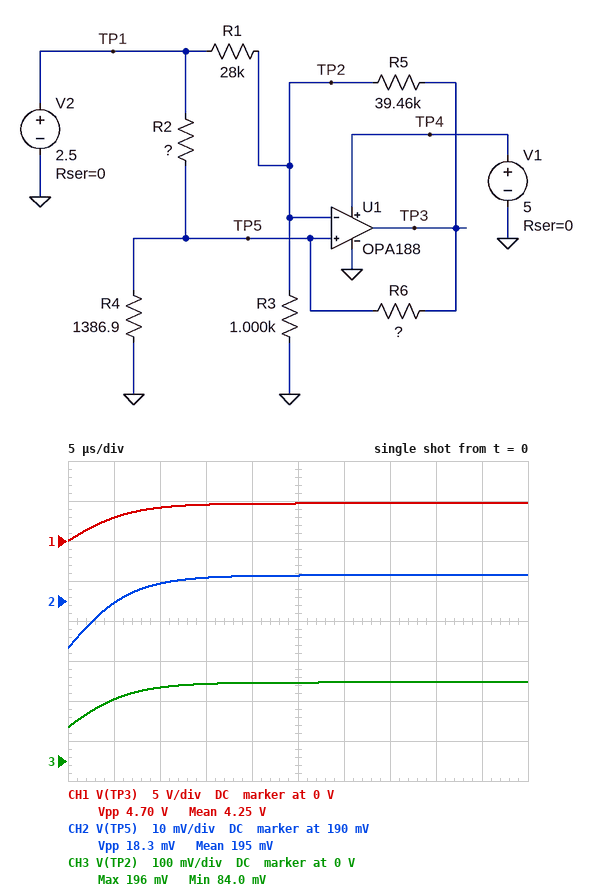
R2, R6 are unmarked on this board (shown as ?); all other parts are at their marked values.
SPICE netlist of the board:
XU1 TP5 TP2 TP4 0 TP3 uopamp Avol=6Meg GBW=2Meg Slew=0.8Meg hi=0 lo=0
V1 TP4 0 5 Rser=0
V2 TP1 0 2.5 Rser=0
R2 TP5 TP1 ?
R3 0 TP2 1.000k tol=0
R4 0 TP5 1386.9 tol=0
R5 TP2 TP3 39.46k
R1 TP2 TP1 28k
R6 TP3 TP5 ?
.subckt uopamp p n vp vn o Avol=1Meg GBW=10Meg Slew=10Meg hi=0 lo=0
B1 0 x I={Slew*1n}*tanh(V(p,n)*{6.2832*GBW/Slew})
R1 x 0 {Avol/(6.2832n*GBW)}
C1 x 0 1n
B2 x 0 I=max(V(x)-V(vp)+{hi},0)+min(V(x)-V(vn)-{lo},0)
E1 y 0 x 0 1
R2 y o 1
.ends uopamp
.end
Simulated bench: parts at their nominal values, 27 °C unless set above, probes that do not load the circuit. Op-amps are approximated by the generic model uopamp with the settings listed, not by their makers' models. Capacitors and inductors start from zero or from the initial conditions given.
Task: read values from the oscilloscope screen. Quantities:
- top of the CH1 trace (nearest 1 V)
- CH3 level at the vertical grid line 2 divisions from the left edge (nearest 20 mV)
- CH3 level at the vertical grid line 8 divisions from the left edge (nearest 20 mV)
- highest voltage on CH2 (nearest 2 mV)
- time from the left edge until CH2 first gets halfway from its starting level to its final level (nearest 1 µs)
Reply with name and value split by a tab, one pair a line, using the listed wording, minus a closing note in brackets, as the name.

top of the CH1 trace	5 V
CH3 level at the vertical grid line 2 divisions from the left edge	180 mV
CH3 level at the vertical grid line 8 divisions from the left edge	200 mV
highest voltage on CH2	196 mV
time from the left edge until CH2 first gets halfway from its starting level to its final level	4 µs
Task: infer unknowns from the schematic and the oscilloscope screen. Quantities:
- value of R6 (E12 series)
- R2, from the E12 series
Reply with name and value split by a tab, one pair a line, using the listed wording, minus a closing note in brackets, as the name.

value of R6	330 kΩ
R2, from the E12 series	18 kΩ
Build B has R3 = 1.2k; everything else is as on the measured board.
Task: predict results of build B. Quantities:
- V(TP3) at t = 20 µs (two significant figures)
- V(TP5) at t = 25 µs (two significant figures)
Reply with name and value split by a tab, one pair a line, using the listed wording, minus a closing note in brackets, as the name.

V(TP3) at t = 20 µs	3.2 V
V(TP5) at t = 25 µs	190 mV
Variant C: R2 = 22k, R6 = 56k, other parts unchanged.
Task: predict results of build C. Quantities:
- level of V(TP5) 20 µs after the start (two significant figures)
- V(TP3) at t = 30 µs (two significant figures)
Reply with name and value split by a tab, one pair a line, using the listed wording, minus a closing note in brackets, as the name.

level of V(TP5) 20 µs after the start	260 mV
V(TP3) at t = 30 µs	5.0 V
